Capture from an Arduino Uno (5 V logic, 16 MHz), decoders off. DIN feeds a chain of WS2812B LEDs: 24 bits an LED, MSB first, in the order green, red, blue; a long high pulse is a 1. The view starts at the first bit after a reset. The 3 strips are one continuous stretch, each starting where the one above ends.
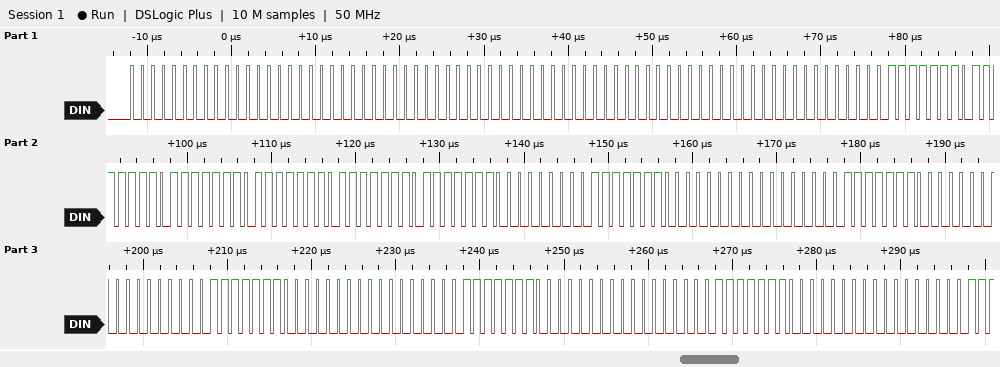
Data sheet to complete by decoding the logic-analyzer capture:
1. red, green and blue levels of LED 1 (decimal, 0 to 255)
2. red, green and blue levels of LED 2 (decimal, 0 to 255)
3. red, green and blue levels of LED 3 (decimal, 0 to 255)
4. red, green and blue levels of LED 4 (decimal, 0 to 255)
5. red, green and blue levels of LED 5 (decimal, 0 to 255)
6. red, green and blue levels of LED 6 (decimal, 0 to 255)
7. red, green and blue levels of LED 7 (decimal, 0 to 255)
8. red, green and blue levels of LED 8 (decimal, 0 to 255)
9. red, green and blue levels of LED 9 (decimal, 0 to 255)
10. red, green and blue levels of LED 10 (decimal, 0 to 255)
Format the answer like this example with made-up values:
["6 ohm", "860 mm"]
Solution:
["0, 0, 0", "0, 0, 0", "0, 0, 0", "254, 254, 254", "254, 254, 254", "254, 0, 0", "254, 0, 0", "254, 0, 0", "254, 0, 0", "254, 0, 0"]
